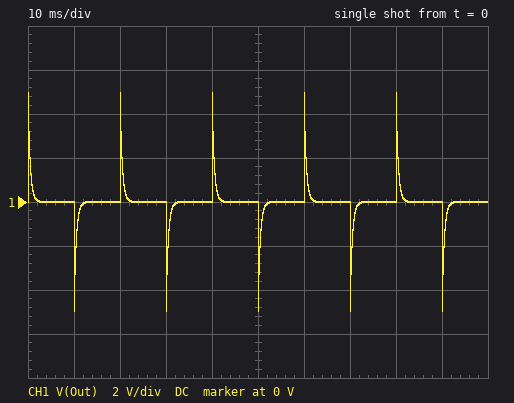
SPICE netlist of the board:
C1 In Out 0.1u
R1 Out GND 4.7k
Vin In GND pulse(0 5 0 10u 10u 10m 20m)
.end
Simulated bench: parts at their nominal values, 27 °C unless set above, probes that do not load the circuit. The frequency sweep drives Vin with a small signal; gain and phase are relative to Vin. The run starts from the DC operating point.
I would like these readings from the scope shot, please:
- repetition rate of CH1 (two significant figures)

50 Hz
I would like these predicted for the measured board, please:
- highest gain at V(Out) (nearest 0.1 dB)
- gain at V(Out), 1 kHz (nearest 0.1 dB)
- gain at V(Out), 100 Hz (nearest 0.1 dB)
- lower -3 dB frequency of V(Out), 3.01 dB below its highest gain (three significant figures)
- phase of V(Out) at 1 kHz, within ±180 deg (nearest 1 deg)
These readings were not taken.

0 dB
-0.5 dB
-11.0 dB
339 Hz
19 deg
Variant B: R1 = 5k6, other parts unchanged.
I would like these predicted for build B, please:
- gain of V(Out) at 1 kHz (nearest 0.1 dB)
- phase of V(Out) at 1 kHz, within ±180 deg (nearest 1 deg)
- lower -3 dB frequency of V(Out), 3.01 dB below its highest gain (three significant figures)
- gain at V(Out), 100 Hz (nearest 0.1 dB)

-0.3 dB
16 deg
284 Hz
-9.6 dB
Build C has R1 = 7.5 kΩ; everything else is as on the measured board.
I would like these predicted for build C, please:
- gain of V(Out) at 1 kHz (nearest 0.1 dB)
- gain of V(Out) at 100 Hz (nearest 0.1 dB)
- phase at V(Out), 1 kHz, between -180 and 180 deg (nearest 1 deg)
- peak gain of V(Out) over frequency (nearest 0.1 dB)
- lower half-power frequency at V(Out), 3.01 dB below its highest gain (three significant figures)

-0.2 dB
-7.4 dB
12 deg
0 dB
212 Hz
